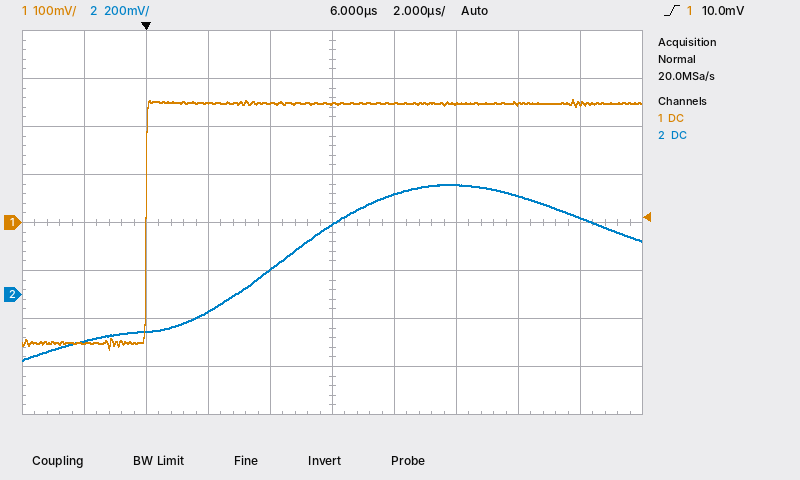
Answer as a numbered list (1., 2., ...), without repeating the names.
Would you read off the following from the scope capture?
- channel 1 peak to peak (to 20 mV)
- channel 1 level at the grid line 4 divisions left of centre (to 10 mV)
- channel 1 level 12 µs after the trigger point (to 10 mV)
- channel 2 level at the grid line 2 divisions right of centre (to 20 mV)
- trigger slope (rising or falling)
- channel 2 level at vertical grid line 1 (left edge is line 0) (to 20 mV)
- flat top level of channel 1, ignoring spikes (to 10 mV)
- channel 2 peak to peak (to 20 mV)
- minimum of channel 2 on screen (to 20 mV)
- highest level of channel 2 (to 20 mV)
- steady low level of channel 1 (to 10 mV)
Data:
1. 520 mV
2. -250 mV
3. 250 mV
4. 460 mV
5. rising
6. -200 mV
7. 250 mV
8. 740 mV
9. -280 mV
10. 460 mV
11. -250 mV
